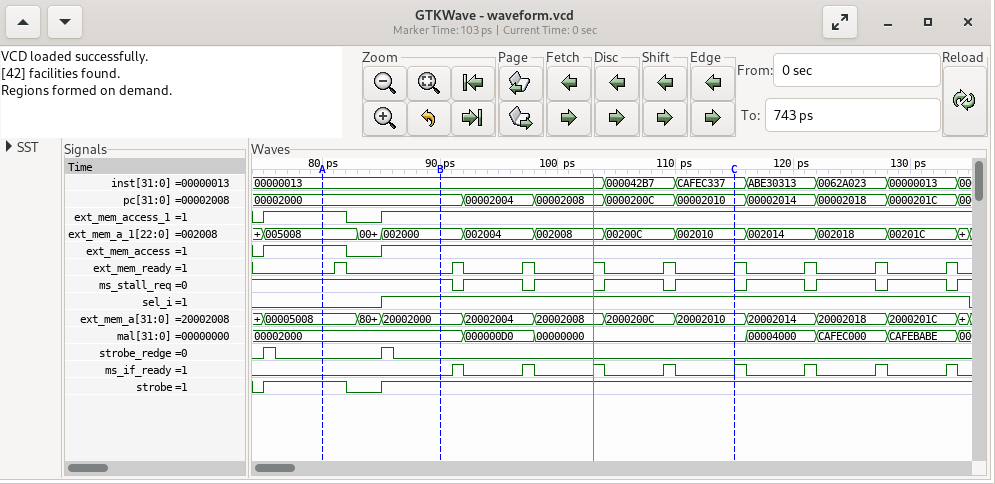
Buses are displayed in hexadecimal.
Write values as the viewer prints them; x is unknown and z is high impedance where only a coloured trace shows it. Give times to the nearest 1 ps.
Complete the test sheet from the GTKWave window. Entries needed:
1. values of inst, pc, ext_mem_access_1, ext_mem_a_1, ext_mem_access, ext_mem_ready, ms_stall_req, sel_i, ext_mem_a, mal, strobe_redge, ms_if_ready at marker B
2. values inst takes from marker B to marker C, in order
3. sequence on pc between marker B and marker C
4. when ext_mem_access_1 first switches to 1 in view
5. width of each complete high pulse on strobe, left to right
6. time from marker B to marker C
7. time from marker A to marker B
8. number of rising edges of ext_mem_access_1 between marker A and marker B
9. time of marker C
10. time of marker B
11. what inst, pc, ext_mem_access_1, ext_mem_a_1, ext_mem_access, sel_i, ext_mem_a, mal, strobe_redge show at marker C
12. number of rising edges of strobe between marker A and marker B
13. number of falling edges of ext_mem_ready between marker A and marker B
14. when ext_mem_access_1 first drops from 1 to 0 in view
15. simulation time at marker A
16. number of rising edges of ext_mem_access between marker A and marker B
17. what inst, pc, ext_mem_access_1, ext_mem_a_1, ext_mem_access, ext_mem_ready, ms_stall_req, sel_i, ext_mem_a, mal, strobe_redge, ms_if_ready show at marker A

inst=00000013, pc=00002000, ext_mem_access_1=1, ext_mem_a_1=002000, ext_mem_access=1, ext_mem_ready=0, ms_stall_req=1, sel_i=1, ext_mem_a=20002000, mal=00002000, strobe_redge=0, ms_if_ready=0
00000013, 000042B7, CAFEC337
00002000, 00002004, 00002008, 0000200C, 00002010
75 ps
7 ps
25 ps
10 ps
1
115 ps
90 ps
inst=CAFEC337, pc=00002010, ext_mem_access_1=1, ext_mem_a_1=002010, ext_mem_access=1, sel_i=1, ext_mem_a=20002010, mal=00000000, strobe_redge=0
1
1
82 ps
80 ps
1
inst=00000013, pc=00002000, ext_mem_access_1=1, ext_mem_a_1=005008, ext_mem_access=1, ext_mem_ready=0, ms_stall_req=1, sel_i=0, ext_mem_a=00005008, mal=00002000, strobe_redge=0, ms_if_ready=0
